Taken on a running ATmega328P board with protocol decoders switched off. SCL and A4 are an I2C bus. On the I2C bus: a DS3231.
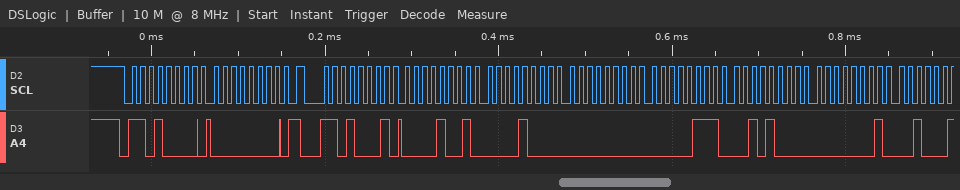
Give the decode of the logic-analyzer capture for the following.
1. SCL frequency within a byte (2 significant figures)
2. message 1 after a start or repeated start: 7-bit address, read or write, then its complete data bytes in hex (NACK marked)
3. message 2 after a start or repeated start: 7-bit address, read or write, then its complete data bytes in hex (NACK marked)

100 kHz
0x68 write: 00
0x68 read: 09 08 00 07 28 01
